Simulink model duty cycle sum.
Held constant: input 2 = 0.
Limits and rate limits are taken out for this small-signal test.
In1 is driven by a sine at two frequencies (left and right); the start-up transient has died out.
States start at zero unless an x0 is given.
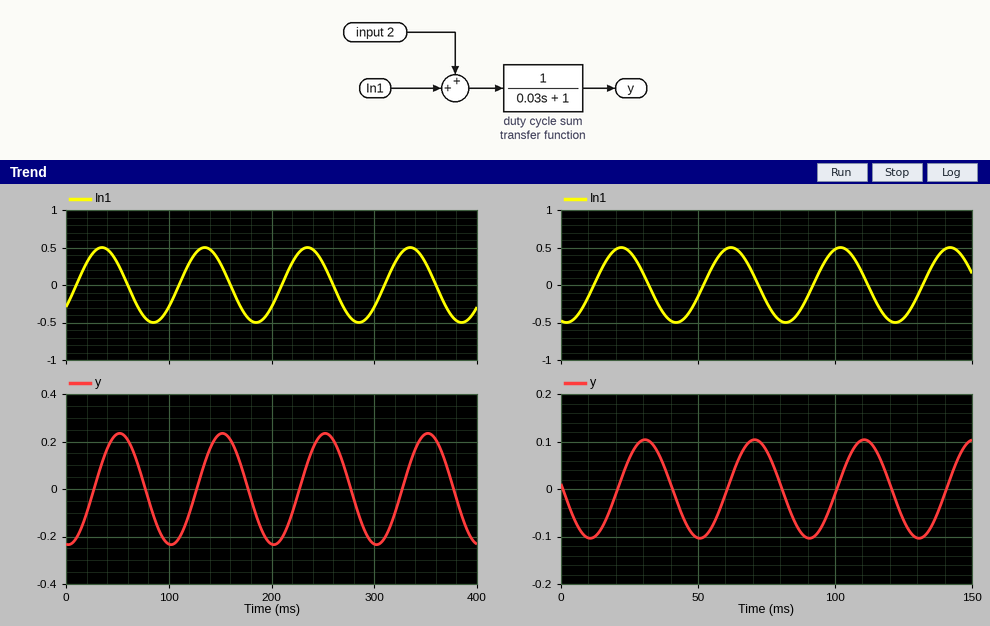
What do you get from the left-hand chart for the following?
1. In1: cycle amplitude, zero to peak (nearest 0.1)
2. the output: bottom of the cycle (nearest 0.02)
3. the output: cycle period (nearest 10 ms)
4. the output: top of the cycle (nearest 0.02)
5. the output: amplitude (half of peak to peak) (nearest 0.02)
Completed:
0.5
-0.24
100 ms
0.24
0.24
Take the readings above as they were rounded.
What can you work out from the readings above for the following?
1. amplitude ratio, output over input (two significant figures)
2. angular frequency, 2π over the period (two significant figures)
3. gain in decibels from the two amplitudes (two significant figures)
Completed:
0.48
0.063 rad/ms
-6.4 dB
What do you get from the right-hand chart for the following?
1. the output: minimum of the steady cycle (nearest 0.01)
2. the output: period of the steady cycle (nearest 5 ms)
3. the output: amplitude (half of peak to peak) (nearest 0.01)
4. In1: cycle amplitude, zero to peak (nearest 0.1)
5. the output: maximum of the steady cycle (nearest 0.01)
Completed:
-0.10
40 ms
0.10
0.5
0.10
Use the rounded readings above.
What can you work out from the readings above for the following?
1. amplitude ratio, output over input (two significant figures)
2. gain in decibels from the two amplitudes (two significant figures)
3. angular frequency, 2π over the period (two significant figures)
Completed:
0.20
-14 dB
0.16 rad/ms
